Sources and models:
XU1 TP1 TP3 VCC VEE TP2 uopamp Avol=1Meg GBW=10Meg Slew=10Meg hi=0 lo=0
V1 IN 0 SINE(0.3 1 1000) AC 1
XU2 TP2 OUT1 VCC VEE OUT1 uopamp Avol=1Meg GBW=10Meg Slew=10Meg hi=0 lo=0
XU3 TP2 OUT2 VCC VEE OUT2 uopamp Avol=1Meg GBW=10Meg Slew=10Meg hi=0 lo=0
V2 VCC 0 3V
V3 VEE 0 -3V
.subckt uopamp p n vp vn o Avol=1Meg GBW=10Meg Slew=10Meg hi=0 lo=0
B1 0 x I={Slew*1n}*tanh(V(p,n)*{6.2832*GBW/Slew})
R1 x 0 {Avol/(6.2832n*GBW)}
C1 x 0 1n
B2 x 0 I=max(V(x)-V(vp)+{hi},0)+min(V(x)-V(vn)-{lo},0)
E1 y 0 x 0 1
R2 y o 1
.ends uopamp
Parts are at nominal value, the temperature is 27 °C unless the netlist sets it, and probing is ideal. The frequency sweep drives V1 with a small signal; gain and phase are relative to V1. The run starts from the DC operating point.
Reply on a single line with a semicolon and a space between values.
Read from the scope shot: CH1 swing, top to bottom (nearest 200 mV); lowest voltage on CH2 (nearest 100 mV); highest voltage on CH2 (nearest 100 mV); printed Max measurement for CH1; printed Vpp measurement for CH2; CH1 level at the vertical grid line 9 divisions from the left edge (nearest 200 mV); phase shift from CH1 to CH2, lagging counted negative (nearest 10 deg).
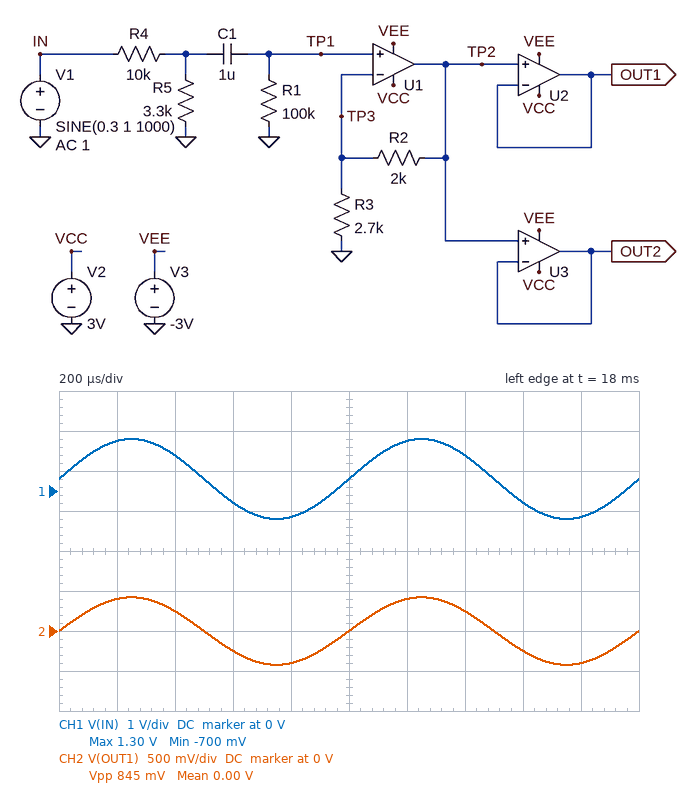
2.0 V; -400 mV; 400 mV; 1.30 V; 845 mV; -600 mV; 0 deg
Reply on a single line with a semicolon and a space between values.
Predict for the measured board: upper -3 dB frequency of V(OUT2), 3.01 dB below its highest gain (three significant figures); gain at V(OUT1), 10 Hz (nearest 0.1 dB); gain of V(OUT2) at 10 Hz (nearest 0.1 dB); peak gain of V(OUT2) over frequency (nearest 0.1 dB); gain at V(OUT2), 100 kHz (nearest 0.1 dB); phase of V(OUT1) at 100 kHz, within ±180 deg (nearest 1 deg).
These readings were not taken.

4.62 MHz; -7.6 dB; -7.6 dB; -7.5 dB; -7.5 dB; -2 deg
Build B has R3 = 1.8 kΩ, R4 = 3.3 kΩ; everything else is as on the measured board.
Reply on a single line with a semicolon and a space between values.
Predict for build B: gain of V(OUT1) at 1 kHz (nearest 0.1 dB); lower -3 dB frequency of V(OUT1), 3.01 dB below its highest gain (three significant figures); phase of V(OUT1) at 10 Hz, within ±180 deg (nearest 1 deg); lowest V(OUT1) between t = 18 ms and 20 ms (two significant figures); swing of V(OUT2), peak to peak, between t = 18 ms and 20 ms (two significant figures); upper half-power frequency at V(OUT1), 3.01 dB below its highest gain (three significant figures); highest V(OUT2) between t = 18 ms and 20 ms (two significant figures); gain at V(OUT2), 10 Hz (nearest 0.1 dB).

0.3 dB; 1.57 Hz; 9 deg; -1.0 V; 2.1 V; 4.02 MHz; 1.0 V; 0.2 dB
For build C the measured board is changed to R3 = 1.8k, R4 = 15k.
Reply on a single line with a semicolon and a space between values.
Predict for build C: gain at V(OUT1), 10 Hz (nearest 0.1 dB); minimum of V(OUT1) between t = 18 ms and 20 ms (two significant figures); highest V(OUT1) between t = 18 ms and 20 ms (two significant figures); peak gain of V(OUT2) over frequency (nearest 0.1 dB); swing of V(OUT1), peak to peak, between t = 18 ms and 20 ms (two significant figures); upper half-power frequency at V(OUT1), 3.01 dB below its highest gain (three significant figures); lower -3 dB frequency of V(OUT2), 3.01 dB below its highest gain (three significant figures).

-8.7 dB; -370 mV; 370 mV; -8.6 dB; 740 mV; 4.02 MHz; 1.55 Hz
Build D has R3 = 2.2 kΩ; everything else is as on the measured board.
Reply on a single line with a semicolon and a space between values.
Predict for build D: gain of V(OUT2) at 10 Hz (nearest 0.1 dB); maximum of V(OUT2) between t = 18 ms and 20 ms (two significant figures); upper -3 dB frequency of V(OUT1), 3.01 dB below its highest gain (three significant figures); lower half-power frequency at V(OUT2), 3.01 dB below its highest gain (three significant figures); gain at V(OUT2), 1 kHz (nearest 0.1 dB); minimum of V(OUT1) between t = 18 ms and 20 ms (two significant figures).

-6.8 dB; 460 mV; 4.33 MHz; 1.55 Hz; -6.7 dB; -460 mV
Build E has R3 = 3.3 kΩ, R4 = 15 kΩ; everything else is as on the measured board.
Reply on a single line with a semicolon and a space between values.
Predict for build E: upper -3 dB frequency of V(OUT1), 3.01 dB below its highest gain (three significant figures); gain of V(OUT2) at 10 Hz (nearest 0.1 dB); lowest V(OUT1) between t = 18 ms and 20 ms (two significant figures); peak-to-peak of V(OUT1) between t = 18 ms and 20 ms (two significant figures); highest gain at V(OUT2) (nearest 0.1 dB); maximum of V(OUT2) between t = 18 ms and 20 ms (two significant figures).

4.88 MHz; -11.1 dB; -280 mV; 560 mV; -11.0 dB; 280 mV
